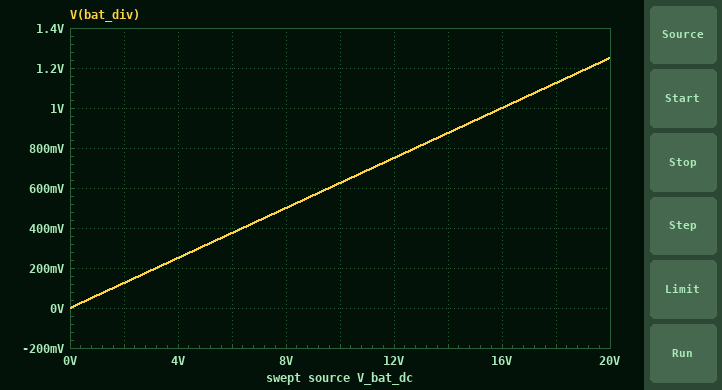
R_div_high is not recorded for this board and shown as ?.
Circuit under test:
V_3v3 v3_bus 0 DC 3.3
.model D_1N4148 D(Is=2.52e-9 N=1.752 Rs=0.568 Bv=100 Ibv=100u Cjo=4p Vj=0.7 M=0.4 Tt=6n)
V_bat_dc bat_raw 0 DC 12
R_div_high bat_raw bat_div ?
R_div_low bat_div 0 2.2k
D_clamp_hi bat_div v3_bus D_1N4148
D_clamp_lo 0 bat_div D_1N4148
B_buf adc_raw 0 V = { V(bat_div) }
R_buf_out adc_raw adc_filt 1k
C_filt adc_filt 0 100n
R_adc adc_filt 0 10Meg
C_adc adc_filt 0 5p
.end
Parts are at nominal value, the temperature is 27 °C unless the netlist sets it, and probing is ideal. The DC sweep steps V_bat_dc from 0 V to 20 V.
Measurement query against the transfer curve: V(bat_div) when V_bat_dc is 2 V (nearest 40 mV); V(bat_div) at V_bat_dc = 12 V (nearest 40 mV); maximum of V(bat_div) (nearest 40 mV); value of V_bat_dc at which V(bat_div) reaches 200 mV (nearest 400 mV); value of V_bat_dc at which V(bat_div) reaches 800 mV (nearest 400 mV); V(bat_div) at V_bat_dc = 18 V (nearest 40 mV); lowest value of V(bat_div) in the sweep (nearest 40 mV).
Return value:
120 mV
760 mV
1.24 V
3.2 V
12.8 V
1.12 V
0 V
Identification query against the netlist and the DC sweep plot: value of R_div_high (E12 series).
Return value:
33 kΩ
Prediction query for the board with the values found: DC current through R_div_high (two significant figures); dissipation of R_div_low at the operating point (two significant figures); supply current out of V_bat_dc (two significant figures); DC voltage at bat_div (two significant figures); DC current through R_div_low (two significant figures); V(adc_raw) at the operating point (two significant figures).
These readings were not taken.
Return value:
340 µA
260 µW
340 µA
750 mV
340 µA
750 mV
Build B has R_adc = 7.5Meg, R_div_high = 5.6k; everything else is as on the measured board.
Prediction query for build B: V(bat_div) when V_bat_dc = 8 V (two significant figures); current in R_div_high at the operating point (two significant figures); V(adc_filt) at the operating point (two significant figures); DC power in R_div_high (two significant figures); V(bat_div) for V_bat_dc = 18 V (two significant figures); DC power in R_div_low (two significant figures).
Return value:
2.3 V
1.5 mA
3.4 V
13 mW
3.9 V
5.2 mW
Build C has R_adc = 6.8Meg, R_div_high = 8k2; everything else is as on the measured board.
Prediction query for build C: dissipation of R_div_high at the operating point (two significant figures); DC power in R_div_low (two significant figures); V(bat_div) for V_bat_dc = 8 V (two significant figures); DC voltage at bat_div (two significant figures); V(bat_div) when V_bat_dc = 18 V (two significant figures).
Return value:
11 mW
2.9 mW
1.7 V
2.5 V
3.7 V
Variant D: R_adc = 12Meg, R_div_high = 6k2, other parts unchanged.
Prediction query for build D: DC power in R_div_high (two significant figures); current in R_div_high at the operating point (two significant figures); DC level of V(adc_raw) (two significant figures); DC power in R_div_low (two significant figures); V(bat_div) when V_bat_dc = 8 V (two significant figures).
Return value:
13 mW
1.4 mA
3.1 V
4.5 mW
2.1 V
